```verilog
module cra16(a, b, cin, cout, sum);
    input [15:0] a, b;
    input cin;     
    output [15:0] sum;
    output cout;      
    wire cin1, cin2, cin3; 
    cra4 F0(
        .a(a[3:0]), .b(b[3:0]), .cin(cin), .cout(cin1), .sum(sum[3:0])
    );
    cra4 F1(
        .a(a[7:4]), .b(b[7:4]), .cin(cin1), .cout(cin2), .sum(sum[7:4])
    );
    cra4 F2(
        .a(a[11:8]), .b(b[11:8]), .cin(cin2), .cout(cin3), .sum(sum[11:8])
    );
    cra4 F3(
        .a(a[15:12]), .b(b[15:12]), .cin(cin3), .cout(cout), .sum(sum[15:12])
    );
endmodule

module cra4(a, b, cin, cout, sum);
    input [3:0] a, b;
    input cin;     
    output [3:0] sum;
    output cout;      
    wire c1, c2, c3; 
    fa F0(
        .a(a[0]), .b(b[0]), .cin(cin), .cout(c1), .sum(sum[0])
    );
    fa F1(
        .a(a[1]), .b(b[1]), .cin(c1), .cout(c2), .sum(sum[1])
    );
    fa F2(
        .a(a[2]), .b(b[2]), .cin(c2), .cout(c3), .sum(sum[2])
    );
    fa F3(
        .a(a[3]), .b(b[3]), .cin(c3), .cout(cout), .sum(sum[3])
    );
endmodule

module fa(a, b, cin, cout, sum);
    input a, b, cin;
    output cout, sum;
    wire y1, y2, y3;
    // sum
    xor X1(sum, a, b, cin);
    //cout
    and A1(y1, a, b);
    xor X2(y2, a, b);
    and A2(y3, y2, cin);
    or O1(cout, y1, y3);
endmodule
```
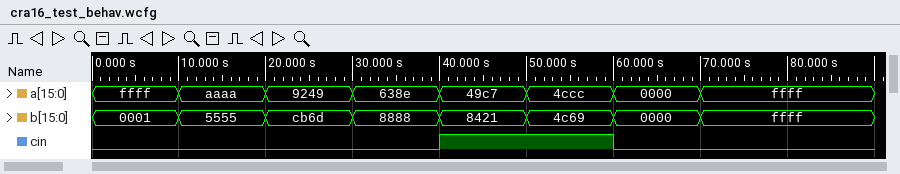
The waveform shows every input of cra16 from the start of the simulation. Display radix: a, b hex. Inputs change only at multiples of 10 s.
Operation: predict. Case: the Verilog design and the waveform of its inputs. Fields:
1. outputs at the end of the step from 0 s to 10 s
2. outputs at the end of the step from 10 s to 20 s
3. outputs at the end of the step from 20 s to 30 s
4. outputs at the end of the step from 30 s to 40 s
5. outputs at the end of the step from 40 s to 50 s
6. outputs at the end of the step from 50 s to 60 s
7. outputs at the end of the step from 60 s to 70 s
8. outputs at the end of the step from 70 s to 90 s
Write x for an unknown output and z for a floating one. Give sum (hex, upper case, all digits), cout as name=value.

sum=0000, cout=1
sum=FFFF, cout=0
sum=5DB6, cout=1
sum=EC16, cout=0
sum=CDE9, cout=0
sum=9936, cout=0
sum=0000, cout=0
sum=FFFE, cout=1
